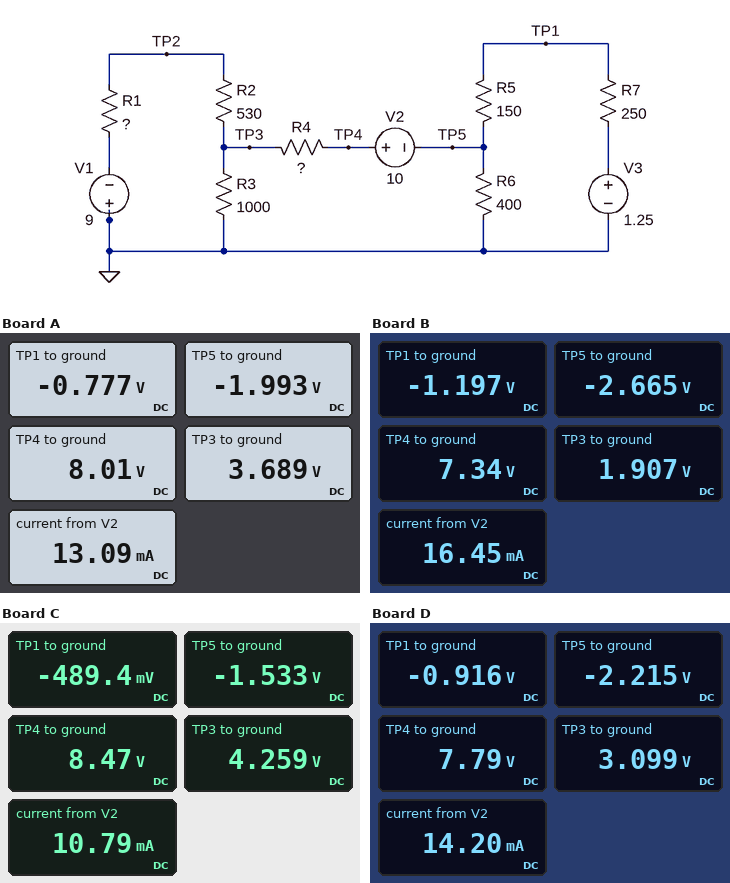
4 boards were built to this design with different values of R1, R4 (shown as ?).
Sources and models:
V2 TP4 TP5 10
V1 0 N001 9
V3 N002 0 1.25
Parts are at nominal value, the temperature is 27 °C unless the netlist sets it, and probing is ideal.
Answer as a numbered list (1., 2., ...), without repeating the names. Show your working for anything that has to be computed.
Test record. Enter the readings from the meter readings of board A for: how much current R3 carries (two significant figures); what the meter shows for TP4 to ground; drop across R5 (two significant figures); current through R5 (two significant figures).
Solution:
1. (3.689 V) / 1 kΩ = 3.7 mA
2. 8.01 V
3. -777 mV - (-1.993 V) = 1.2 V
4. (-777 mV - (-1.993 V)) / 150 Ω = 8.1 mA
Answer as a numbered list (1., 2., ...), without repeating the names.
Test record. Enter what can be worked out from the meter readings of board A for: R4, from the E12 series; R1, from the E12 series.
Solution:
1. 330 Ω
2. 820 Ω
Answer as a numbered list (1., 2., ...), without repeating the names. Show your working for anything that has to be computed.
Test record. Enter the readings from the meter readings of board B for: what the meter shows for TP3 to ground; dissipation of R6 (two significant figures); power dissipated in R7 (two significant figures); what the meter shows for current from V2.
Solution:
1. 1.907 V
2. (0 V - (-2.665 V))^2 / 400 Ω = 18 mW
3. (1.25 V - (-1.197 V))^2 / 250 Ω = 24 mW
4. 16.45 mA
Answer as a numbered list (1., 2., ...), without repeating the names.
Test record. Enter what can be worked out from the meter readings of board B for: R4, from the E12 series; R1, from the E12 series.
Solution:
1. 330 Ω
2. 220 Ω
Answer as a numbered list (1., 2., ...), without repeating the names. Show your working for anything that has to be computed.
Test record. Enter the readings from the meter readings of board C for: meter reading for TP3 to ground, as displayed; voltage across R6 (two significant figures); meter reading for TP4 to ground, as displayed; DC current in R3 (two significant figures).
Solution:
1. 4.259 V
2. 0 V - (-1.533 V) = 1.5 V
3. 8.47 V
4. (4.259 V) / 1 kΩ = 4.3 mA
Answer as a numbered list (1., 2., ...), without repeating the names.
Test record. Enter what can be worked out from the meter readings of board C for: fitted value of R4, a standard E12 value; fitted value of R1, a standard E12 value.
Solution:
1. 390 Ω
2. 1.5 kΩ
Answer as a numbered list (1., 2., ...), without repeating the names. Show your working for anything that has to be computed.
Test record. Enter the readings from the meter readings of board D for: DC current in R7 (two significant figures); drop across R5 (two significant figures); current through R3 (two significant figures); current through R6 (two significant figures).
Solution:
1. (1.25 V - (-916 mV)) / 250 Ω = 8.7 mA
2. -916 mV - (-2.215 V) = 1.3 V
3. (3.099 V) / 1 kΩ = 3.1 mA
4. (0 V - (-2.215 V)) / 400 Ω = 5.5 mA
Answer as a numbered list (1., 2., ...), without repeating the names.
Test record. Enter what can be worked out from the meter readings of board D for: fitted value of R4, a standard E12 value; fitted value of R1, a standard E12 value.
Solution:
1. 330 Ω
2. 560 Ω
